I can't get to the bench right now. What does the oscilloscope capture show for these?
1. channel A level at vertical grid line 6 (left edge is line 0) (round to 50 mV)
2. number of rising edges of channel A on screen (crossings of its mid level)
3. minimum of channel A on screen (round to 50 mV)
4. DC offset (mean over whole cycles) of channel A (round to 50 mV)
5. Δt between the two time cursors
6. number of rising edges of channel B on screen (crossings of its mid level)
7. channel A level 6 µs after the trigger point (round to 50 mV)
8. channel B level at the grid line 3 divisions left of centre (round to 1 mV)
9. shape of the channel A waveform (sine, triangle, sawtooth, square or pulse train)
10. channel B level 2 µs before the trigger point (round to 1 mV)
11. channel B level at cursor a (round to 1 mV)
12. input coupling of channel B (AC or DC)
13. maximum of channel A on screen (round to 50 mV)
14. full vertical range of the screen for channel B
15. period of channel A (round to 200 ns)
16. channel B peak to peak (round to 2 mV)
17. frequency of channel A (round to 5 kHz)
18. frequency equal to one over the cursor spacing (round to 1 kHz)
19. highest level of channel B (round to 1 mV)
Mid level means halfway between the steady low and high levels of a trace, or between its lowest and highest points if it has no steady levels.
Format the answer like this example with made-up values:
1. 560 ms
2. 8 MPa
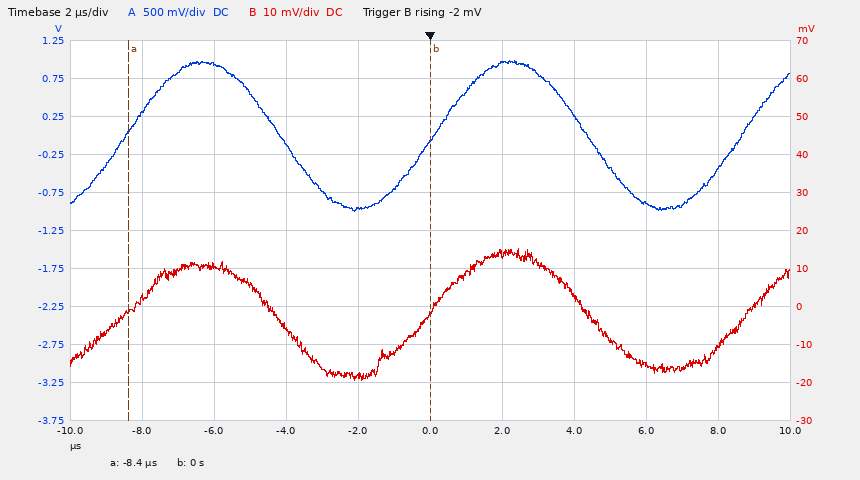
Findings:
1. 950 mV
2. 3
3. -1.00 V
4. 0 mV
5. 8.4 µs
6. 3
7. -900 mV
8. 11 mV
9. sine
10. -18 mV
11. -1 mV
12. DC
13. 1.00 V
14. 100 mV
15. 8.6 µs
16. 34 mV
17. 115 kHz
18. 119 kHz
19. 15 mV
